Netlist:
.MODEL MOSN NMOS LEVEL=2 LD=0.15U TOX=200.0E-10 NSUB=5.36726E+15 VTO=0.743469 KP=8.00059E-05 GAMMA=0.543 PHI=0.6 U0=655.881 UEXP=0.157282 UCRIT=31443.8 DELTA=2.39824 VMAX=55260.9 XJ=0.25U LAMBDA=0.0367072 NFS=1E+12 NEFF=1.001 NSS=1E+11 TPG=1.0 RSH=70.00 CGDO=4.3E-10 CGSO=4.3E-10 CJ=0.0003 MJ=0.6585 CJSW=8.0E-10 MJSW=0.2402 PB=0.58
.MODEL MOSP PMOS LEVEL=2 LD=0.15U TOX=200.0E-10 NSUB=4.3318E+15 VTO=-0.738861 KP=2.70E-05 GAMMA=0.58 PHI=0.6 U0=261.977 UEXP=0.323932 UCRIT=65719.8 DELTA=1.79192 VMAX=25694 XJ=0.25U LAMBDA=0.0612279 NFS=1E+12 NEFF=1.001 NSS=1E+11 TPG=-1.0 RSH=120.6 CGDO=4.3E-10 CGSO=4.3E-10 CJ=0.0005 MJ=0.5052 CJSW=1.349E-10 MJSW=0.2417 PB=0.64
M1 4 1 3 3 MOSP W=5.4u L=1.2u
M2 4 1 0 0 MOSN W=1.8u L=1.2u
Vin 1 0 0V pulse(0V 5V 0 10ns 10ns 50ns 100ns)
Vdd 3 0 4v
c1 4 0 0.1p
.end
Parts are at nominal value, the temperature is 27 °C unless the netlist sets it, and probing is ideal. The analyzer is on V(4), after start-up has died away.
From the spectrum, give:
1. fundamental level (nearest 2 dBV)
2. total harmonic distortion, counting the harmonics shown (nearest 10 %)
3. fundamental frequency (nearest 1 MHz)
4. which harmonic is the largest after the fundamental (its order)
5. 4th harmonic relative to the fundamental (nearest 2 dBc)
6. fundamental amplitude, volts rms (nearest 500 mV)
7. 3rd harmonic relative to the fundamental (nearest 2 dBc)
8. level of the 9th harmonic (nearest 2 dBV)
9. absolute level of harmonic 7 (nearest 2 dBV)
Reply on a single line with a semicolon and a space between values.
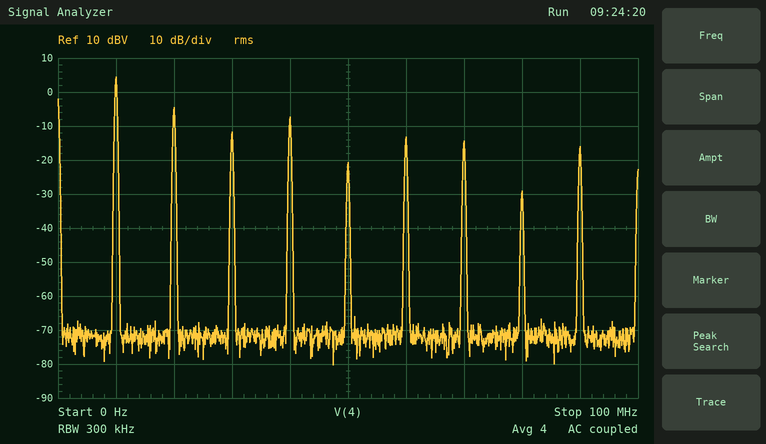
4 dBV; 50 %; 10 MHz; 2; -12 dBc; 1.5 V; -16 dBc; -16 dBV; -14 dBV
